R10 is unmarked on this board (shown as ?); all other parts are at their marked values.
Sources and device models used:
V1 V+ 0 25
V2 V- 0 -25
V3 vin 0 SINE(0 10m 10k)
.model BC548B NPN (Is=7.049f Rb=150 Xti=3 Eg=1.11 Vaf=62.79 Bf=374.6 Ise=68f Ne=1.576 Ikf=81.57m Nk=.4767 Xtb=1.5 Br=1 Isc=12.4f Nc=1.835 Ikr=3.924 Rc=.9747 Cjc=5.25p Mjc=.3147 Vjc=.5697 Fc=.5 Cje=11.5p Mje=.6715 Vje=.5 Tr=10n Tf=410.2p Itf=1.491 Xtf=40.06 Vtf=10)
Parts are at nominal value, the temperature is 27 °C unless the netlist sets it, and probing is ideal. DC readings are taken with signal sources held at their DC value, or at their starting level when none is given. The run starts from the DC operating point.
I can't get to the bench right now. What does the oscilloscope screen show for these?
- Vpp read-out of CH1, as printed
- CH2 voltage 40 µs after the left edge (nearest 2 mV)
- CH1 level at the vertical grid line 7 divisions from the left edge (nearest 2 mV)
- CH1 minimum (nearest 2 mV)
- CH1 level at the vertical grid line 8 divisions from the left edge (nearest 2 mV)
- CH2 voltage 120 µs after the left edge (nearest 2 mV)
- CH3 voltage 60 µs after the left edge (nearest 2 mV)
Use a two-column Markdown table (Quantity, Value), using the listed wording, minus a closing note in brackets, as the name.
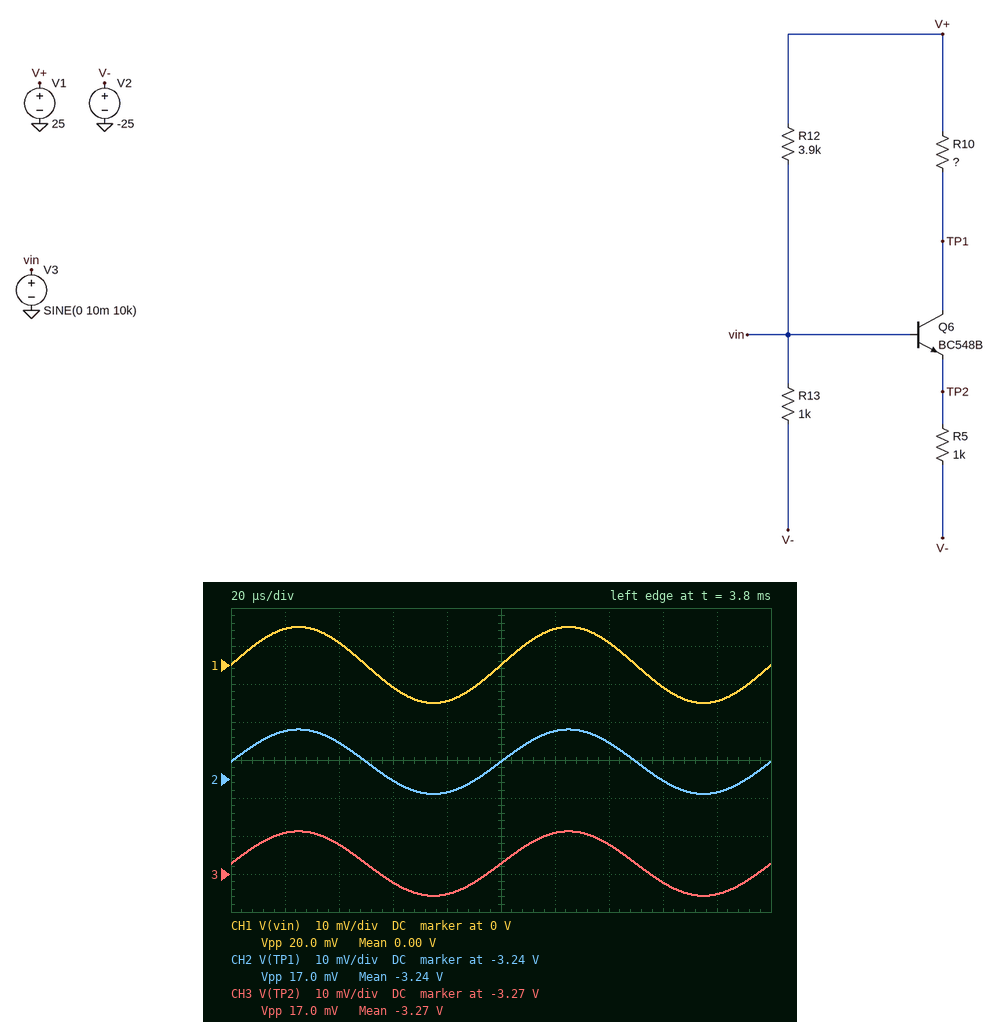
| Quantity | Value |
|---|---|
| Vpp read-out of CH1, as printed | 20.0 mV |
| CH2 voltage 40 µs after the left edge | -3.230 V |
| CH1 level at the vertical grid line 7 divisions from the left edge | 6 mV |
| CH1 minimum | -10 mV |
| CH1 level at the vertical grid line 8 divisions from the left edge | -6 mV |
| CH2 voltage 120 µs after the left edge | -3.228 V |
| CH3 voltage 60 µs after the left edge | -3.272 V |
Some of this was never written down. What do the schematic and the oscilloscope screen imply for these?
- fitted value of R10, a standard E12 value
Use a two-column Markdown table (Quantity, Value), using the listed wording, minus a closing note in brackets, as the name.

| Quantity | Value |
|---|---|
| fitted value of R10, a standard E12 value | 5.6 kΩ |
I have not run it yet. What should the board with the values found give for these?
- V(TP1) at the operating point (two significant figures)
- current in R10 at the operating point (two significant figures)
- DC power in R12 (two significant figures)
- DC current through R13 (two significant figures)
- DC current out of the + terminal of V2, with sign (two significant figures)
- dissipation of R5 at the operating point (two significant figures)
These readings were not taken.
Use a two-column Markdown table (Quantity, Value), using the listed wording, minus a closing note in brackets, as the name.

| Quantity | Value |
|---|---|
| V(TP1) at the operating point | -3.2 V |
| current in R10 at the operating point | 5.0 mA |
| DC power in R12 | 160 mW |
| DC current through R13 | 25 mA |
| DC current out of the + terminal of V2, with sign | -47 mA |
| dissipation of R5 at the operating point | 470 mW |
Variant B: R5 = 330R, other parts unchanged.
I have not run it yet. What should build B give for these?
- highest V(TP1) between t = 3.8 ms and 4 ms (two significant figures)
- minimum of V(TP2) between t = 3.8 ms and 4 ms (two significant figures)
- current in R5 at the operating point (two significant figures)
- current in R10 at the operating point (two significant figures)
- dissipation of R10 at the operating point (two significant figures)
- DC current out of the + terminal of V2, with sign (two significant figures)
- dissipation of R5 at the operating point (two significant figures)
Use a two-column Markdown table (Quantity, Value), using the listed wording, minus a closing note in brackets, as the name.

| Quantity | Value |
|---|---|
| highest V(TP1) between t = 3.8 ms and 4 ms | -7.7 V |
| minimum of V(TP2) between t = 3.8 ms and 4 ms | -7.8 V |
| current in R5 at the operating point | 52 mA |
| current in R10 at the operating point | 5.8 mA |
| dissipation of R10 at the operating point | 190 mW |
| DC current out of the + terminal of V2, with sign | -77 mA |
| dissipation of R5 at the operating point | 900 mW |
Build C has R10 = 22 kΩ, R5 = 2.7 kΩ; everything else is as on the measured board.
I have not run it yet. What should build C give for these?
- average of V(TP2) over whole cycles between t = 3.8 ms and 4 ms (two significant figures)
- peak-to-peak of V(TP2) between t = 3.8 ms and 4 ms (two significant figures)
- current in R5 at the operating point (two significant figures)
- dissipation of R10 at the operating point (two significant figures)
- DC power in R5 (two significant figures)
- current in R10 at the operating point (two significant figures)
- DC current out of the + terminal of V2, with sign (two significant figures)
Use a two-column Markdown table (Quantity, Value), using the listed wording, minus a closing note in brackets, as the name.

| Quantity | Value |
|---|---|
| average of V(TP2) over whole cycles between t = 3.8 ms and 4 ms | -1.8 V |
| peak-to-peak of V(TP2) between t = 3.8 ms and 4 ms | 19 mV |
| current in R5 at the operating point | 8.6 mA |
| dissipation of R10 at the operating point | 33 mW |
| DC power in R5 | 200 mW |
| current in R10 at the operating point | 1.2 mA |
| DC current out of the + terminal of V2, with sign | -34 mA |
